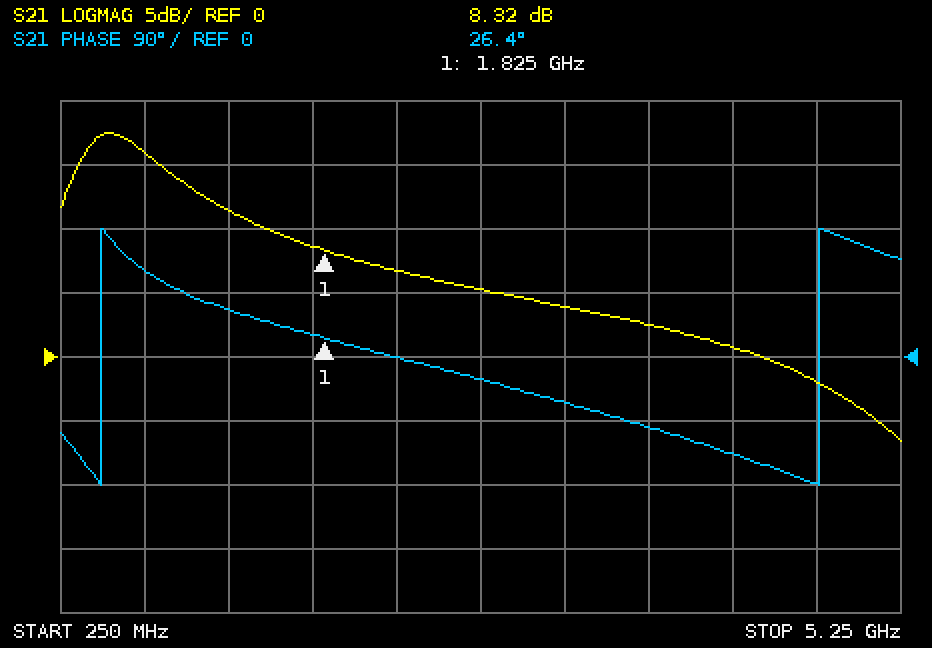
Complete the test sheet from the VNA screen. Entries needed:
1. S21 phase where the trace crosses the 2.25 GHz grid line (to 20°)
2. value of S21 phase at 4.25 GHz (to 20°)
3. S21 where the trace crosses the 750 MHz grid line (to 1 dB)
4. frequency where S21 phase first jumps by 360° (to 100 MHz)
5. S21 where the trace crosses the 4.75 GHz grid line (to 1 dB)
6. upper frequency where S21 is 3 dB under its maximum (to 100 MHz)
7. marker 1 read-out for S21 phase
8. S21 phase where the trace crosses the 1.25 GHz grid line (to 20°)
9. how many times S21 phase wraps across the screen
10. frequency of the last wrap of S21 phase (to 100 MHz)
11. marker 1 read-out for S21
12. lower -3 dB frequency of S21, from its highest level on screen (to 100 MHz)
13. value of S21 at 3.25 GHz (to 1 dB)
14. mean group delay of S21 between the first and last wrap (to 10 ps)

0°
-140°
16 dB
500 MHz
-2 dB
900 MHz
26.4°
60°
2
4.8 GHz
8.32 dB
300 MHz
4 dB
230 ps
